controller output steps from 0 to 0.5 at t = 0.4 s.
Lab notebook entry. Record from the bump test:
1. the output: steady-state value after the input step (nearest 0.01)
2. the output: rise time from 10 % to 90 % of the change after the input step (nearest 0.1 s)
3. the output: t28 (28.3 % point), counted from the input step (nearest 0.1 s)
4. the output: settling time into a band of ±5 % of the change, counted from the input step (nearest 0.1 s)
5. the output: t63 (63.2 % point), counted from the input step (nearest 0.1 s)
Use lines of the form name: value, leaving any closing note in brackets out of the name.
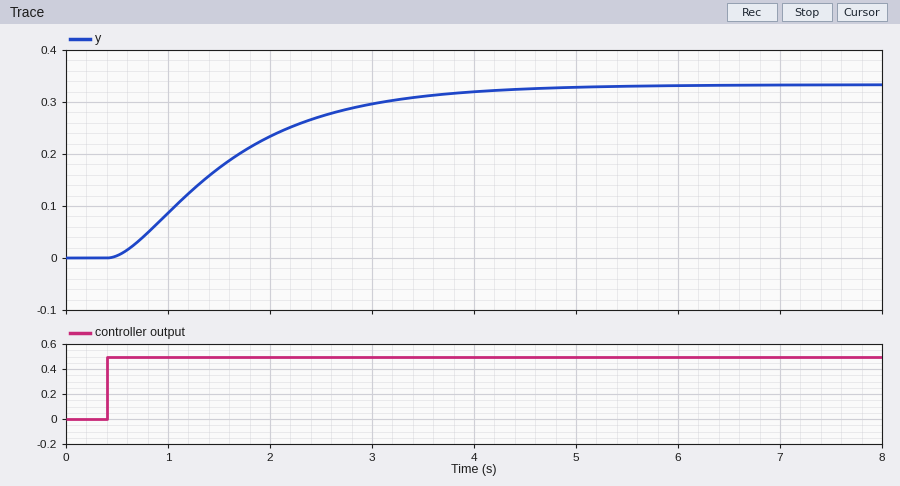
the output: steady-state value after the input step: 0.33
the output: rise time from 10 % to 90 % of the change after the input step: 2.4 s
the output: t28 (28.3 % point), counted from the input step: 0.6 s
the output: settling time into a band of ±5 % of the change, counted from the input step: 3.4 s
the output: t63 (63.2 % point), counted from the input step: 1.4 s
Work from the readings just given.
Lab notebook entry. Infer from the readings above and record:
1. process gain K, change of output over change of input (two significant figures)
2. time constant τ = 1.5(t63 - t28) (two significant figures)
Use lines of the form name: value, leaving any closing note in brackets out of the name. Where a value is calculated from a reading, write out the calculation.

process gain K, change of output over change of input: (0.33 - 0) / 0.5 = 0.66
time constant τ = 1.5(t63 - t28): 1.5 × (1.4 - 0.6) = 1.2 s
